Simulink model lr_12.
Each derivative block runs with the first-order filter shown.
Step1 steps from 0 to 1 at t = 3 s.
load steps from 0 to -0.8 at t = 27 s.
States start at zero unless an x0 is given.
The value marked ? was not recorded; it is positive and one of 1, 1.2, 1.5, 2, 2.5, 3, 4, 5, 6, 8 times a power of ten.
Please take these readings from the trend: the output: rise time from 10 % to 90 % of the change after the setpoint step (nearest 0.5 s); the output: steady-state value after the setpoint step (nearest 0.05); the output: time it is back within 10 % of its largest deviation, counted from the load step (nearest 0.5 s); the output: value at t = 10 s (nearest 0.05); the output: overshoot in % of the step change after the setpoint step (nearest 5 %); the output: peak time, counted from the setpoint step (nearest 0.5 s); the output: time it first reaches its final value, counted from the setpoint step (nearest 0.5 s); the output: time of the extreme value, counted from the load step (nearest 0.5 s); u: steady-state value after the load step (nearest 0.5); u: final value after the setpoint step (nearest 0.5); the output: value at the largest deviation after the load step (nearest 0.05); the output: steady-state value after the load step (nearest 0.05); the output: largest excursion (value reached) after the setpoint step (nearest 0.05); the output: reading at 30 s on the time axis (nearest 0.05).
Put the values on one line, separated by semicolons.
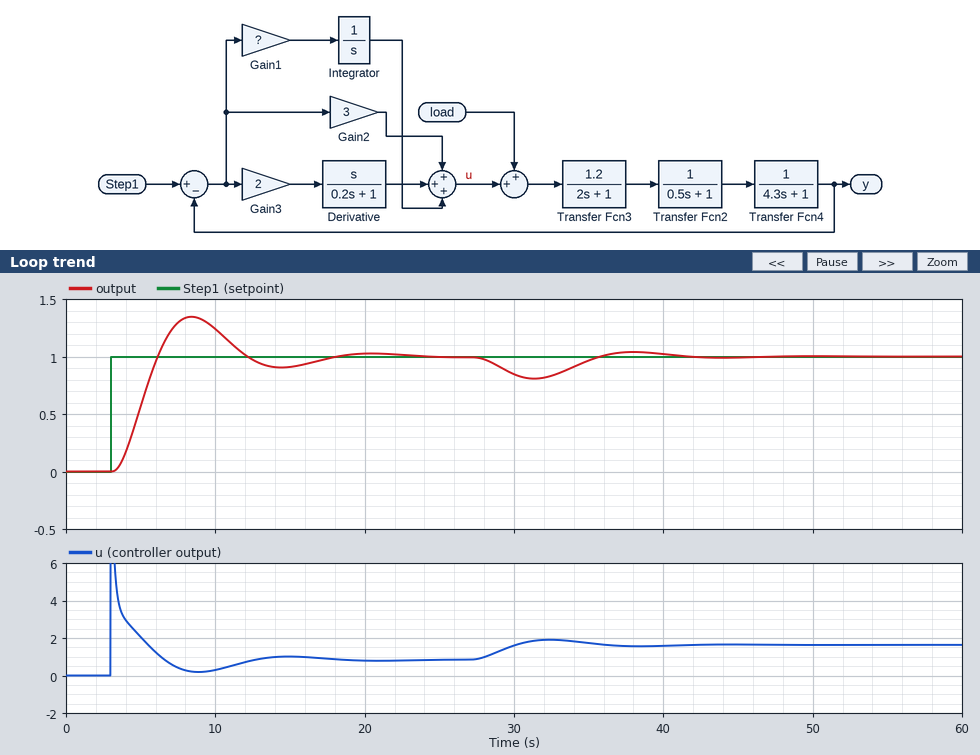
2.0 s; 1.00; 13.0 s; 1.25; 35 %; 5.5 s; 3.0 s; 4.5 s; 1.5; 1.0; 0.80; 1.00; 1.35; 0.85
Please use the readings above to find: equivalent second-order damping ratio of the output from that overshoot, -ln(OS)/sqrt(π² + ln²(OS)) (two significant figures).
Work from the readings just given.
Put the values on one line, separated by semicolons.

0.32
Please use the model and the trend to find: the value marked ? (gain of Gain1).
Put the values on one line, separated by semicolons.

1
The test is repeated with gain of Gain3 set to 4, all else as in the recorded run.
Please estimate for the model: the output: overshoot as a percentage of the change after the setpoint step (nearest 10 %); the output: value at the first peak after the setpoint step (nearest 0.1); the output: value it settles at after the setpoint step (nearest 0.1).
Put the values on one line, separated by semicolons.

20 %; 1.2; 1.0
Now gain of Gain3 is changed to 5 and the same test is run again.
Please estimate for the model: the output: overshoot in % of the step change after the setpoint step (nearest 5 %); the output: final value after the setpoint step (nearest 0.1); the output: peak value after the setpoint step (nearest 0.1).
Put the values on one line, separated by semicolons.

10 %; 1.0; 1.1
